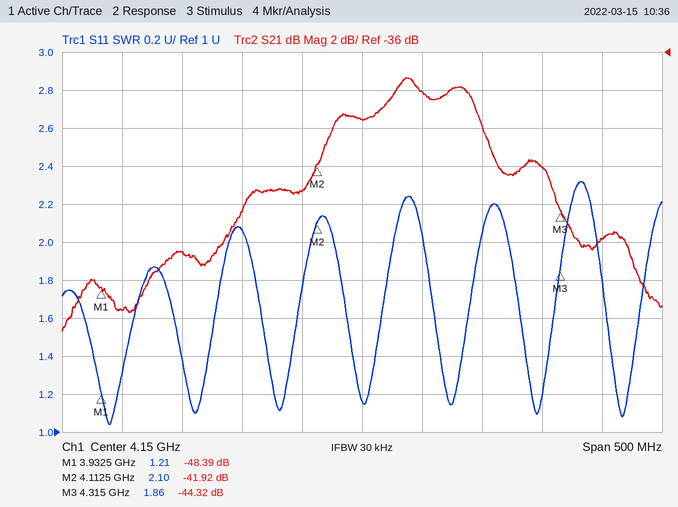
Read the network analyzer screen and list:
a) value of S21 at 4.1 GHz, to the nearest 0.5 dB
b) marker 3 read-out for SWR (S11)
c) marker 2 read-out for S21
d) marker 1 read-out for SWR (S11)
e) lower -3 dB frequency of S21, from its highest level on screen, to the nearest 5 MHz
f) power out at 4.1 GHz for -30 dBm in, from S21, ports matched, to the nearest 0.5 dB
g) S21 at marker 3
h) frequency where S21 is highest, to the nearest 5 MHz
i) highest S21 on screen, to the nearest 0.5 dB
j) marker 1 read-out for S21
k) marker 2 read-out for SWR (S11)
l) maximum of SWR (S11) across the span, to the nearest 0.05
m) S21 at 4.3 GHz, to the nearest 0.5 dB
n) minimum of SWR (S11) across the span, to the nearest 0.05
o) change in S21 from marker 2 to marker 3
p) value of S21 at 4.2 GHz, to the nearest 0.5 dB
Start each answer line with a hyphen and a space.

- -43.5 dB
- 1.86
- -41.92 dB
- 1.21
- 4.125 GHz
- -73.5 dBm
- -44.32 dB
- 4.185 GHz
- -37.5 dB
- -48.39 dB
- 2.10
- 2.30
- -42.0 dB
- 1.05
- -2.40 dB
- -38.0 dB
